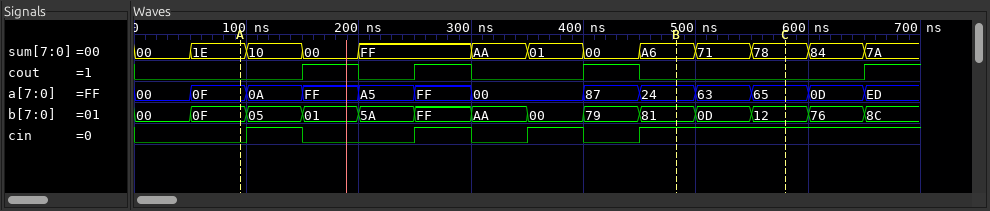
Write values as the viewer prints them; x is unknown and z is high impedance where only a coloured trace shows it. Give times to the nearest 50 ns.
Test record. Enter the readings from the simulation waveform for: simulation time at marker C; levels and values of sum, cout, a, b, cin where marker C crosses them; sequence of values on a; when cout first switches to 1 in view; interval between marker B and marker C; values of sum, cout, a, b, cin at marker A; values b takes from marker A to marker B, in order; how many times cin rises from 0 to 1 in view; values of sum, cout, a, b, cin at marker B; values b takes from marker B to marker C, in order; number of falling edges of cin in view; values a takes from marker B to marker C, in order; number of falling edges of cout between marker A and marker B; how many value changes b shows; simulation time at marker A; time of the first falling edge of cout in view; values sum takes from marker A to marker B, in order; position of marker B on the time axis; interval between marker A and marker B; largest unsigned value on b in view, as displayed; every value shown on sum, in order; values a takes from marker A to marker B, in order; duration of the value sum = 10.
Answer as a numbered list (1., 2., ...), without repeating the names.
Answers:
1. 600 ns
2. sum=78, cout=0, a=65, b=12, cin=1
3. 00, 0F, 0A, FF, A5, FF, 00, 87, 24, 63, 65, 0D, ED
4. 150 ns
5. 100 ns
6. sum=1E, cout=0, a=0F, b=0F, cin=0
7. 0F, 05, 01, 5A, FF, AA, 00, 79, 81
8. 4
9. sum=A6, cout=0, a=24, b=81, cin=1
10. 81, 0D, 12
11. 3
12. 24, 63, 65
13. 3
14. 13
15. 100 ns
16. 200 ns
17. 1E, 10, 00, FF, AA, 01, 00, A6
18. 500 ns
19. 400 ns
20. FF
21. 00, 1E, 10, 00, FF, AA, 01, 00, A6, 71, 78, 84, 7A
22. 0F, 0A, FF, A5, FF, 00, 87, 24
23. 50 ns
